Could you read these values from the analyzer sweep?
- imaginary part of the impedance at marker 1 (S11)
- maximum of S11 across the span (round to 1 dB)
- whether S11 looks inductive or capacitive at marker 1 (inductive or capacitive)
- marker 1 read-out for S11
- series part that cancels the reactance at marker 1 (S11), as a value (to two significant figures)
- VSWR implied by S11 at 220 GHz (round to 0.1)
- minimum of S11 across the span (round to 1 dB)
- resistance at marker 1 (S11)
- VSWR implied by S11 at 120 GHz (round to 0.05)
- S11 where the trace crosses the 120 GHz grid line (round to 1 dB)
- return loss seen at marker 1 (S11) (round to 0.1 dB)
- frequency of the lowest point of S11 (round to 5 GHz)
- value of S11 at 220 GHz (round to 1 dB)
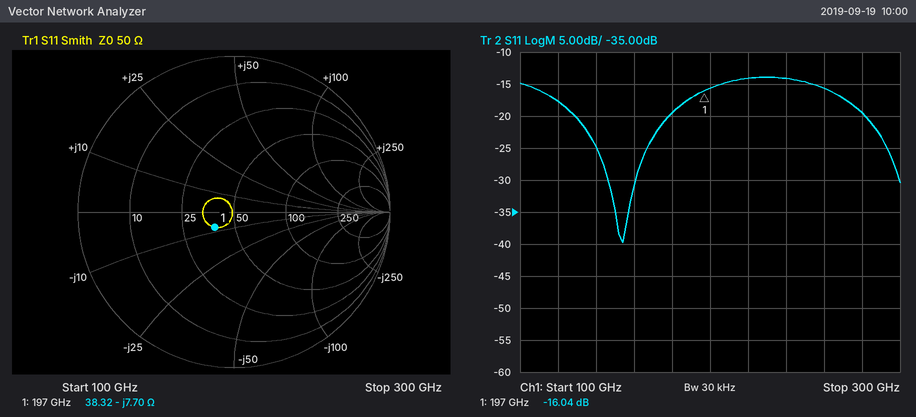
-7.70 Ω
-14 dB
capacitive
-16.04 dB
6.2 pH
1.5
-40 dB
38.32 Ω
1.30
-18 dB
16.0 dB
155 GHz
-14 dB
